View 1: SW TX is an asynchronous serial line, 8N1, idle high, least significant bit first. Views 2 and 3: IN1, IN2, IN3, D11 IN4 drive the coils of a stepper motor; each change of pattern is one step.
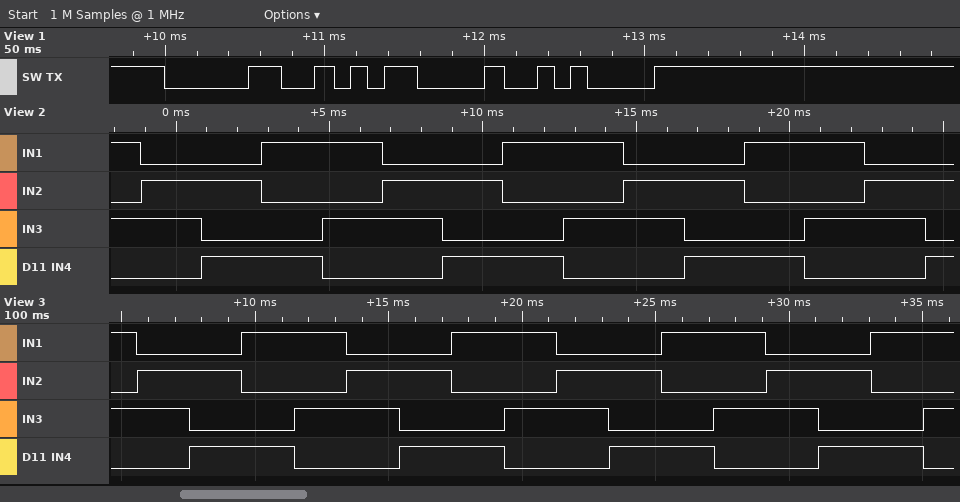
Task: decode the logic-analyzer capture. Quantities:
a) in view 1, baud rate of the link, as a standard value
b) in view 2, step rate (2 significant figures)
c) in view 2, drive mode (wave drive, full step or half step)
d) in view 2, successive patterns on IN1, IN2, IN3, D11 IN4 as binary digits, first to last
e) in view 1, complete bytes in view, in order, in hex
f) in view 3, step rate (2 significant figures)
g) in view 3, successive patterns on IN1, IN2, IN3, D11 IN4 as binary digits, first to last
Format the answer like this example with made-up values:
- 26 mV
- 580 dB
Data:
- 9600 baud
- 510 steps/s
- full step
- 1010 0110 0101 1001 1010 0110 0101 1001 1010 0110 0101 1001 1010 0110 0101
- 30 0D 0A
- 510 steps/s
- 1010 0110 0101 1001 1010 0110 0101 1001 1010 0110 0101 1001 1010 0110 0101 1001 1010
